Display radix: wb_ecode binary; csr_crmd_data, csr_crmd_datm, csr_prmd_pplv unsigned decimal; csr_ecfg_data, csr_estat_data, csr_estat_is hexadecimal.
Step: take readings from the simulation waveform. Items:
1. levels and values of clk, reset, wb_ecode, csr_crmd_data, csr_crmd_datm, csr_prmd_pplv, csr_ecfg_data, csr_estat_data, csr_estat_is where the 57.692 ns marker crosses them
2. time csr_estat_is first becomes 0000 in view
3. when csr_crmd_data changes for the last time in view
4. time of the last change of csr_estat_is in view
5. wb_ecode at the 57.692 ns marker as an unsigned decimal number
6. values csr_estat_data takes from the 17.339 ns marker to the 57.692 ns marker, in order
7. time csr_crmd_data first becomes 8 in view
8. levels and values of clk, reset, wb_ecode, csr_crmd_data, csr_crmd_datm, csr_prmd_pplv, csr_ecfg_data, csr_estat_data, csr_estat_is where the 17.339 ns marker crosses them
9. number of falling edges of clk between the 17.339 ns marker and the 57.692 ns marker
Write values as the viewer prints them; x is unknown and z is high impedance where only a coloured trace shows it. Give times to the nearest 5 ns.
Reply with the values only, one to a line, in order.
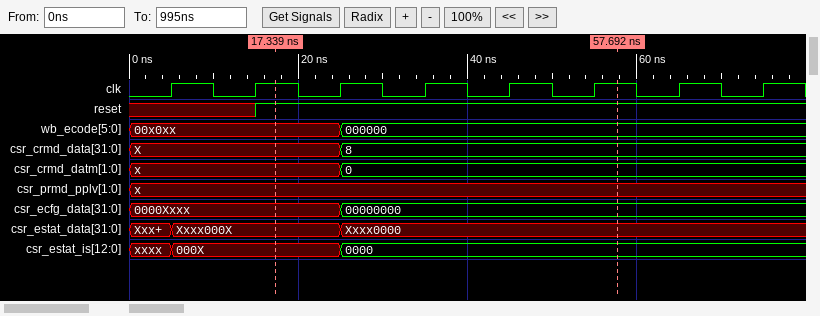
clk=1, reset=1, wb_ecode=000000, csr_crmd_data=8, csr_crmd_datm=0, csr_prmd_pplv=x, csr_ecfg_data=00000000, csr_estat_data=Xxxx0000, csr_estat_is=0000
25 ns
25 ns
25 ns
0
Xxxx000X, Xxxx0000
25 ns
clk=1, reset=1, wb_ecode=00x0xx, csr_crmd_data=X, csr_crmd_datm=x, csr_prmd_pplv=x, csr_ecfg_data=0000Xxxx, csr_estat_data=Xxxx000X, csr_estat_is=000X
4
